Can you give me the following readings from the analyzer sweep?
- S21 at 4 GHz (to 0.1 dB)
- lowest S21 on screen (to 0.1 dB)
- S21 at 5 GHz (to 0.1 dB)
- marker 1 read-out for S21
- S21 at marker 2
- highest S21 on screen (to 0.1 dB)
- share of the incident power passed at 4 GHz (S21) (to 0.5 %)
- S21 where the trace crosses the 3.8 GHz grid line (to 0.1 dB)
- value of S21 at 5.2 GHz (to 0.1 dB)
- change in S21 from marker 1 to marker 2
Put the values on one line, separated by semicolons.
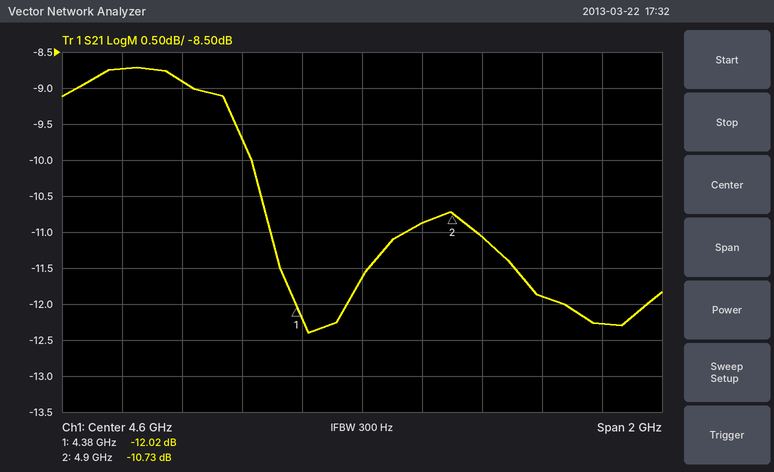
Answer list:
-8.9 dB; -12.4 dB; -11.1 dB; -12.02 dB; -10.73 dB; -8.7 dB; 13.0 %; -8.7 dB; -11.9 dB; 1.29 dB
